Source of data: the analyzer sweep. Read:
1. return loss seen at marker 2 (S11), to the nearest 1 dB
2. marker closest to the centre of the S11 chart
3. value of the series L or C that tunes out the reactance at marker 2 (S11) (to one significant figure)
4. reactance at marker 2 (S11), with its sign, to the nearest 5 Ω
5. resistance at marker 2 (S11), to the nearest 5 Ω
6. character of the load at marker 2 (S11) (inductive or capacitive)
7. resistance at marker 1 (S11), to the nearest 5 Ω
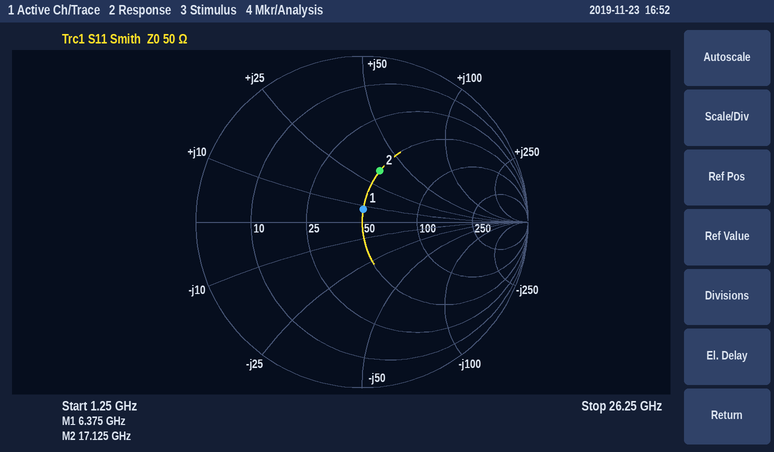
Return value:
10 dB
marker 1
300 fF
+35 Ω
50 Ω
inductive
50 Ω
